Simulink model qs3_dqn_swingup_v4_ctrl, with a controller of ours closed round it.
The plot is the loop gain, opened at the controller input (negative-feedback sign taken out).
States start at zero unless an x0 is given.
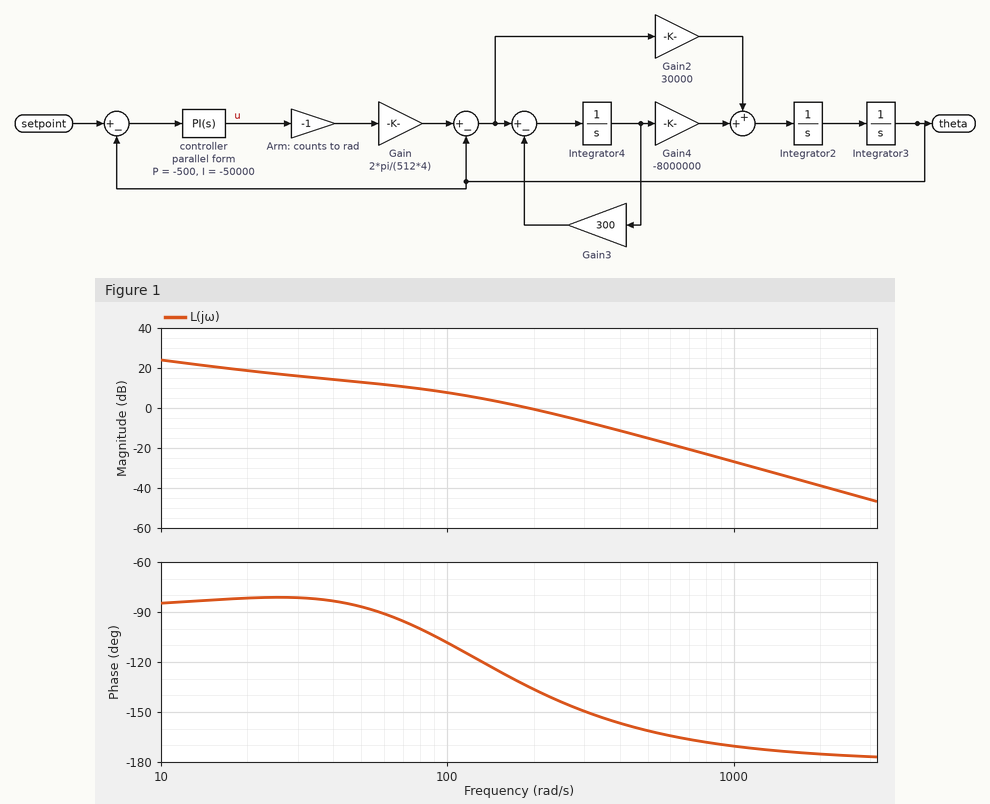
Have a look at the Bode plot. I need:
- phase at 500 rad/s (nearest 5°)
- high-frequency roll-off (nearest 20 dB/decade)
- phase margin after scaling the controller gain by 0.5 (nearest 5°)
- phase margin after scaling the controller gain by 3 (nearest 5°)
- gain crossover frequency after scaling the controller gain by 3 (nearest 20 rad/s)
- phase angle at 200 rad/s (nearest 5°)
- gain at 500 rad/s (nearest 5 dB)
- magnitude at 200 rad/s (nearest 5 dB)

-160°
-40 dB/decade
65°
25°
360 rad/s
-135°
-15 dB
0 dB
